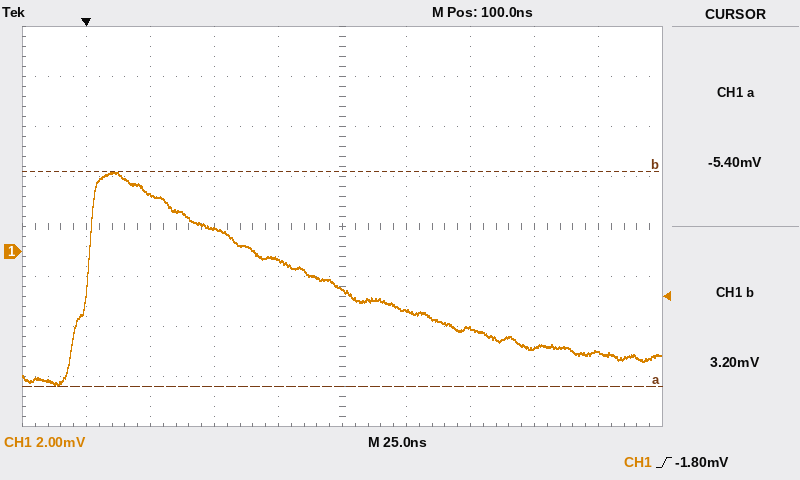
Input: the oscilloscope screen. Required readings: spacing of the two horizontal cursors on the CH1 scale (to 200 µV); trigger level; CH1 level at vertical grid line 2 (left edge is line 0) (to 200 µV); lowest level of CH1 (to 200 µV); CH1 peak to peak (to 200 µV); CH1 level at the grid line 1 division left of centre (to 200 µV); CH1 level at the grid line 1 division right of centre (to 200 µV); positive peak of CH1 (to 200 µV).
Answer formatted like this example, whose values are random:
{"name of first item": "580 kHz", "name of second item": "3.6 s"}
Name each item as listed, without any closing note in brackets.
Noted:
{"spacing of the two horizontal cursors on the CH1 scale": "8.6 mV", "trigger level": "-1.80 mV", "CH1 level at vertical grid line 2 (left edge is line 0)": "2.2 mV", "lowest level of CH1": "-5.4 mV", "CH1 peak to peak": "8.6 mV", "CH1 level at the grid line 1 division left of centre": "-400 µV", "CH1 level at the grid line 1 division right of centre": "-2.4 mV", "positive peak of CH1": "3.2 mV"}
